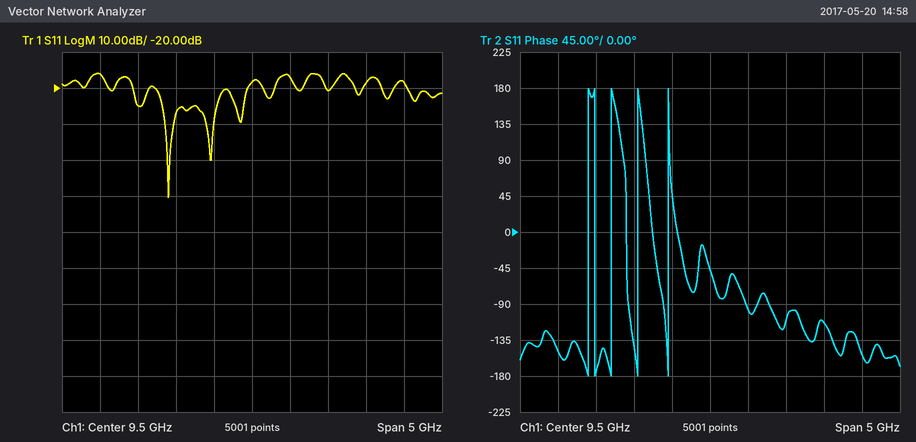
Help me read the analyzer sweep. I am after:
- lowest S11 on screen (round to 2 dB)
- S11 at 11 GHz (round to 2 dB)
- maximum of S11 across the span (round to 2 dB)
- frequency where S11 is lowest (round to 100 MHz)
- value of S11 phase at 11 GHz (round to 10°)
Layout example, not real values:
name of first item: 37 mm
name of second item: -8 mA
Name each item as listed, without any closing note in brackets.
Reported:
lowest S11 on screen: -50 dB
S11 at 11 GHz: -18 dB
maximum of S11 across the span: -16 dB
frequency where S11 is lowest: 8.4 GHz
value of S11 phase at 11 GHz: -110°
